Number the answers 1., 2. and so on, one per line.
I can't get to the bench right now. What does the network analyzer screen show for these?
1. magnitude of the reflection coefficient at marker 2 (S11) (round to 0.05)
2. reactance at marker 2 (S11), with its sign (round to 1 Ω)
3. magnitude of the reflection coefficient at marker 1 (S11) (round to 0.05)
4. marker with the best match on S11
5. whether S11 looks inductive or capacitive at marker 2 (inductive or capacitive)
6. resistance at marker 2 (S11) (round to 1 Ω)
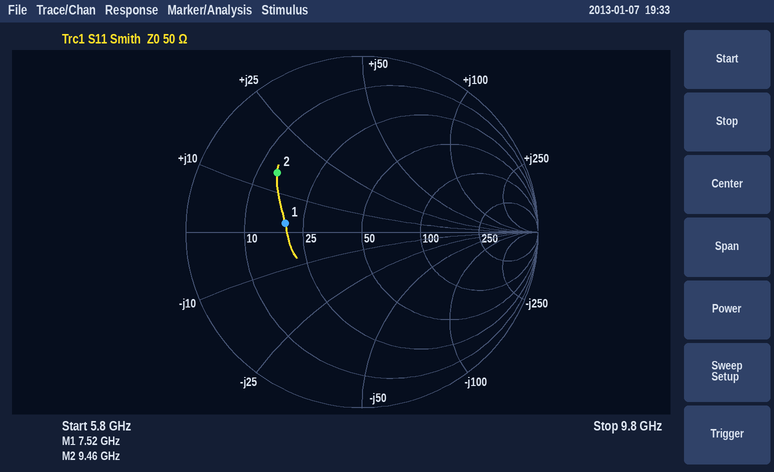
1. 0.60
2. +15 Ω
3. 0.45
4. marker 1
5. inductive
6. 14 Ω
